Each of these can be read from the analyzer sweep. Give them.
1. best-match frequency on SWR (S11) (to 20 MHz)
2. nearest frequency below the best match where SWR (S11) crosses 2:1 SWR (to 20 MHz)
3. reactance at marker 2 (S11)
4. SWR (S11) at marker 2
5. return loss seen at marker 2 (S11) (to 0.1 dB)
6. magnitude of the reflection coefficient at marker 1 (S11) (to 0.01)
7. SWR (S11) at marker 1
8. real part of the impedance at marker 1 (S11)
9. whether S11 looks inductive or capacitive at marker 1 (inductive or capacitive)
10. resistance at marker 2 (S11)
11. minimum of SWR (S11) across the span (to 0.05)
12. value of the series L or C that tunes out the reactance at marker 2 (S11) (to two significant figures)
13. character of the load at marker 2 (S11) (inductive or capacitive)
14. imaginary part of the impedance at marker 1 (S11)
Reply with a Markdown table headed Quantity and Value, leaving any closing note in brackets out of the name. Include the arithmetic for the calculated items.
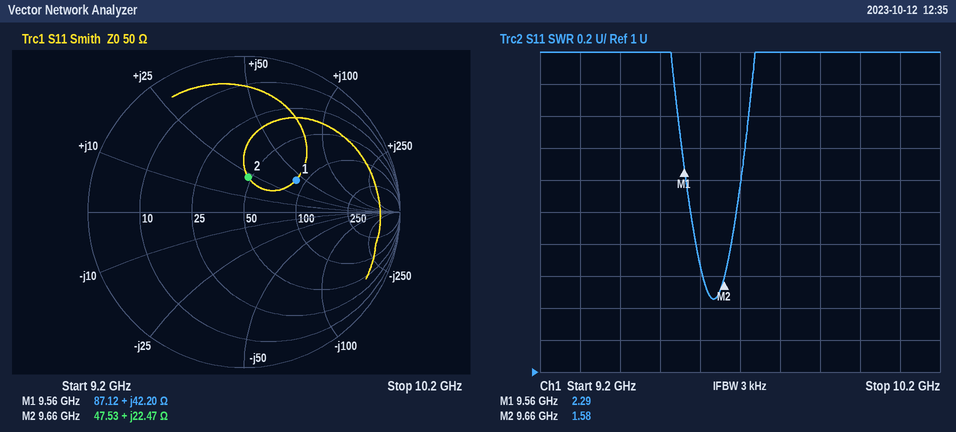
| Quantity | Value |
|---|---|
| best-match frequency on SWR (S11) | 9.64 GHz |
| nearest frequency below the best match where SWR (S11) crosses 2:1 SWR | 9.58 GHz |
| reactance at marker 2 | +22.47 Ω |
| SWR (S11) at marker 2 | 1.58 |
| return loss seen at marker 2 (S11) | 12.9 dB |
| magnitude of the reflection coefficient at marker 1 (S11) | 0.39 |
| SWR (S11) at marker 1 | 2.29 |
| real part of the impedance at marker 1 | 87.12 Ω |
| whether S11 looks inductive or capacitive at marker 1 | inductive |
| resistance at marker 2 | 47.53 Ω |
| minimum of SWR (S11) across the span | 1.45 |
| value of the series L or C that tunes out the reactance at marker 2 (S11) | C = 1/(2π × 9.66 GHz × 22.47 Ω) ≈ 733 fF, so 730 fF to two significant figures |
| character of the load at marker 2 (S11) | inductive |
| imaginary part of the impedance at marker 1 | +42.20 Ω |
